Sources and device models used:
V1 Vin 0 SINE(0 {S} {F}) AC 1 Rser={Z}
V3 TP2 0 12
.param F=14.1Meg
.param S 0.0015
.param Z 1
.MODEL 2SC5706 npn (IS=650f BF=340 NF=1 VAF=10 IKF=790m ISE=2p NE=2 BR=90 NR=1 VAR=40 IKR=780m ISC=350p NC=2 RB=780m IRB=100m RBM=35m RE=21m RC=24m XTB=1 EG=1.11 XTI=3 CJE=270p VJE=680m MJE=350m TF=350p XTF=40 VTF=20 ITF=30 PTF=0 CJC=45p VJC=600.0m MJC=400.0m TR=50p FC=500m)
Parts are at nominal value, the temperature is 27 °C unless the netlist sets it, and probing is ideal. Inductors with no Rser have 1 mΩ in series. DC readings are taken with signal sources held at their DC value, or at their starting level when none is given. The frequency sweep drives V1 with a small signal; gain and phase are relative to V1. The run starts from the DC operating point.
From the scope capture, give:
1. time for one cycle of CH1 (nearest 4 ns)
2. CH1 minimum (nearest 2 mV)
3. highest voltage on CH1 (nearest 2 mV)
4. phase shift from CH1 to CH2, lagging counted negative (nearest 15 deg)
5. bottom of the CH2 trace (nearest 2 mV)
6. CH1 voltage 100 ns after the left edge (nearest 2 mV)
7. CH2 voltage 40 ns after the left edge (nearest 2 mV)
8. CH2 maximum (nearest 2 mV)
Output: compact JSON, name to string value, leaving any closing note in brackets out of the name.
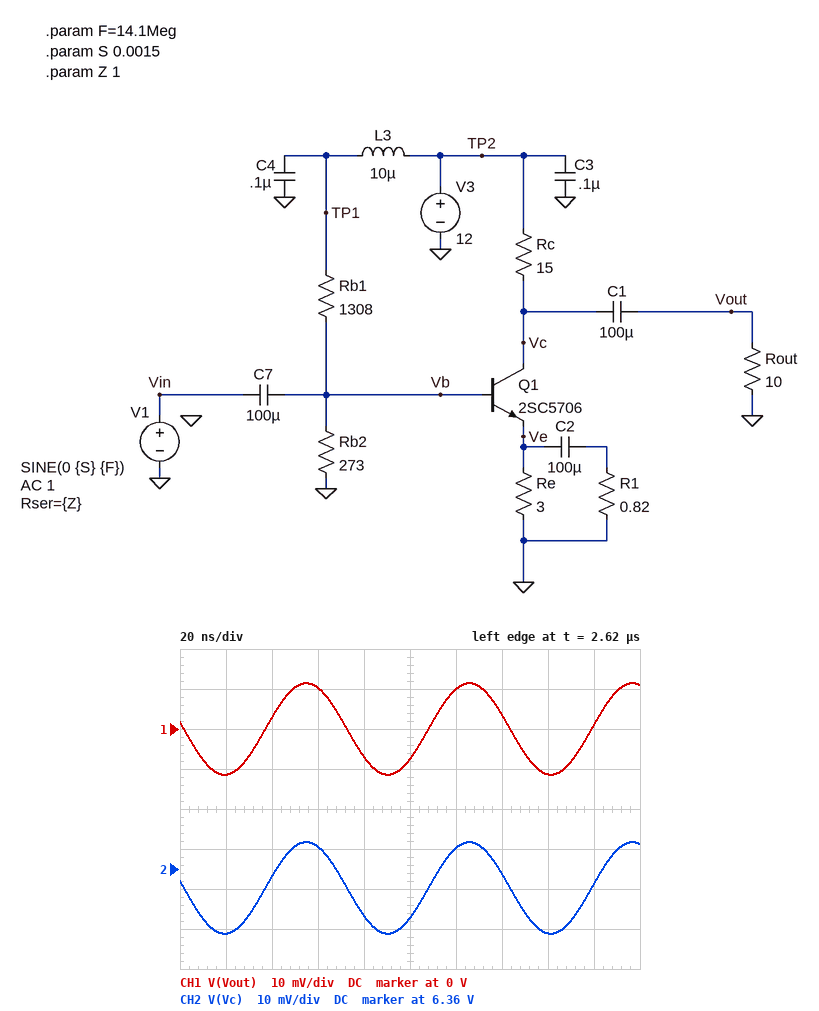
{"time for one cycle of CH1": "72 ns", "CH1 minimum": "-12 mV", "highest voltage on CH1": "12 mV", "phase shift from CH1 to CH2, lagging counted negative": "0 deg", "bottom of the CH2 trace": "6.344 V", "CH1 voltage 100 ns after the left edge": "-8 mV", "CH2 voltage 40 ns after the left edge": "6.358 V", "CH2 maximum": "6.366 V"}
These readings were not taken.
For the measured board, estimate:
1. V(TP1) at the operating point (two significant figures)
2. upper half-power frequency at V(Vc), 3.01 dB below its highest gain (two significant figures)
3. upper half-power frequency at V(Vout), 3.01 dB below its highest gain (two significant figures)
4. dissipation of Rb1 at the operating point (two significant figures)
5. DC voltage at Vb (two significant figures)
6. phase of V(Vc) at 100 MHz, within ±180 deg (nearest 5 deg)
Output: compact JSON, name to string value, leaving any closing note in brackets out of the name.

{"V(TP1) at the operating point": "12 V", "upper half-power frequency at V(Vc), 3.01 dB below its highest gain": "100 MHz", "upper half-power frequency at V(Vout), 3.01 dB below its highest gain": "100 MHz", "dissipation of Rb1 at the operating point": "79 mW", "DC voltage at Vb": "1.8 V", "phase of V(Vc) at 100 MHz, within ±180 deg": "130 deg"}
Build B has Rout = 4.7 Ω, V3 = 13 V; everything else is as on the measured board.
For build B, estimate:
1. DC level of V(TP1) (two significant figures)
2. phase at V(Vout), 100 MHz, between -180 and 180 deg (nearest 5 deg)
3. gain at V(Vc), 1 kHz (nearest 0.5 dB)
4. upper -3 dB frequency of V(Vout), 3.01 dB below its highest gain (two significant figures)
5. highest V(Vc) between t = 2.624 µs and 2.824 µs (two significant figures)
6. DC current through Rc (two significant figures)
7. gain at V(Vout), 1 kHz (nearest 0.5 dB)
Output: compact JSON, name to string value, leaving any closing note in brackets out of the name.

{"DC level of V(TP1)": "13 V", "phase at V(Vout), 100 MHz, between -180 and 180 deg": "135 deg", "gain at V(Vc), 1 kHz": "8.5 dB", "upper -3 dB frequency of V(Vout), 3.01 dB below its highest gain": "110 MHz", "highest V(Vc) between t = 2.624 µs and 2.824 µs": "6.7 V", "DC current through Rc": "420 mA", "gain at V(Vout), 1 kHz": "8.0 dB"}
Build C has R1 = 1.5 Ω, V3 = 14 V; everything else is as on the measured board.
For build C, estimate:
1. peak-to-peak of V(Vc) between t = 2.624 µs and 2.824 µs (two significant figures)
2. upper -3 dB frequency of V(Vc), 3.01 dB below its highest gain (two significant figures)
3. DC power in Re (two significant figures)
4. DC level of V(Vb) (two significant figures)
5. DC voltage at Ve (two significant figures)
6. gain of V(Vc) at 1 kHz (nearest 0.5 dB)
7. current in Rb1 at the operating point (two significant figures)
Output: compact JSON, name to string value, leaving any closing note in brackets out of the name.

{"peak-to-peak of V(Vc) between t = 2.624 µs and 2.824 µs": "16 mV", "upper -3 dB frequency of V(Vc), 3.01 dB below its highest gain": "130 MHz", "DC power in Re": "660 mW", "DC level of V(Vb)": "2.1 V", "DC voltage at Ve": "1.4 V", "gain of V(Vc) at 1 kHz": "12.0 dB", "current in Rb1 at the operating point": "9.1 mA"}
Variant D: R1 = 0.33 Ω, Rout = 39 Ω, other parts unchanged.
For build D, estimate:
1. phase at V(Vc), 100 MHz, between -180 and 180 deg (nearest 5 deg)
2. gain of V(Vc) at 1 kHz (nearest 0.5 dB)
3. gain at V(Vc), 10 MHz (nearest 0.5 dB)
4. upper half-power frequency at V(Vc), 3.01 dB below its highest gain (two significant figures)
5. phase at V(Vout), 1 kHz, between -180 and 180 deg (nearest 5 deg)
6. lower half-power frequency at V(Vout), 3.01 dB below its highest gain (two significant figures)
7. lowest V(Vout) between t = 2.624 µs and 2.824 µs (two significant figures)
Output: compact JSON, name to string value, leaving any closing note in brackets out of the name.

{"phase at V(Vc), 100 MHz, between -180 and 180 deg": "115 deg", "gain of V(Vc) at 1 kHz": "17.5 dB", "gain at V(Vc), 10 MHz": "27.5 dB", "upper half-power frequency at V(Vc), 3.01 dB below its highest gain": "56 MHz", "phase at V(Vout), 1 kHz, between -180 and 180 deg": "-130 deg", "lower half-power frequency at V(Vout), 3.01 dB below its highest gain": "3.4 kHz", "lowest V(Vout) between t = 2.624 µs and 2.824 µs": "-36 mV"}
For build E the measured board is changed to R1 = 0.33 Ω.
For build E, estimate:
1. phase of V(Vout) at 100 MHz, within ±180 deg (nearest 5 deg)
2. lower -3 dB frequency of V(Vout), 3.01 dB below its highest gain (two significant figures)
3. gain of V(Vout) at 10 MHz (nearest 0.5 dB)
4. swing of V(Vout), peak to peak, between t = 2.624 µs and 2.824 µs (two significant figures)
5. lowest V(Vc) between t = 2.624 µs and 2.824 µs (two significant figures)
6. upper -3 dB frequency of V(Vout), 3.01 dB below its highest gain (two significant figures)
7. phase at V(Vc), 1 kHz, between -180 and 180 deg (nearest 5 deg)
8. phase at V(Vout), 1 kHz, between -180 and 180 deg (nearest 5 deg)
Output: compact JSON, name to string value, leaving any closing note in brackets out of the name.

{"phase of V(Vout) at 100 MHz, within ±180 deg": "120 deg", "lower -3 dB frequency of V(Vout), 3.01 dB below its highest gain": "3.5 kHz", "gain of V(Vout) at 10 MHz": "23.0 dB", "swing of V(Vout), peak to peak, between t = 2.624 µs and 2.824 µs": "41 mV", "lowest V(Vc) between t = 2.624 µs and 2.824 µs": "6.3 V", "upper -3 dB frequency of V(Vout), 3.01 dB below its highest gain": "64 MHz", "phase at V(Vc), 1 kHz, between -180 and 180 deg": "-135 deg", "phase at V(Vout), 1 kHz, between -180 and 180 deg": "-125 deg"}
